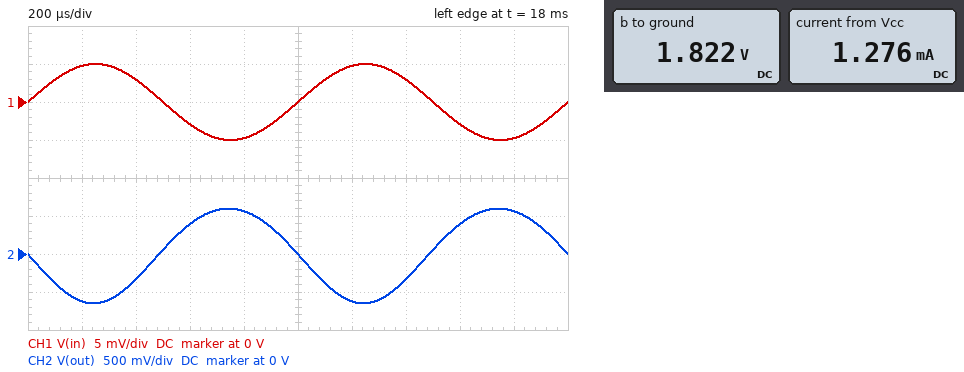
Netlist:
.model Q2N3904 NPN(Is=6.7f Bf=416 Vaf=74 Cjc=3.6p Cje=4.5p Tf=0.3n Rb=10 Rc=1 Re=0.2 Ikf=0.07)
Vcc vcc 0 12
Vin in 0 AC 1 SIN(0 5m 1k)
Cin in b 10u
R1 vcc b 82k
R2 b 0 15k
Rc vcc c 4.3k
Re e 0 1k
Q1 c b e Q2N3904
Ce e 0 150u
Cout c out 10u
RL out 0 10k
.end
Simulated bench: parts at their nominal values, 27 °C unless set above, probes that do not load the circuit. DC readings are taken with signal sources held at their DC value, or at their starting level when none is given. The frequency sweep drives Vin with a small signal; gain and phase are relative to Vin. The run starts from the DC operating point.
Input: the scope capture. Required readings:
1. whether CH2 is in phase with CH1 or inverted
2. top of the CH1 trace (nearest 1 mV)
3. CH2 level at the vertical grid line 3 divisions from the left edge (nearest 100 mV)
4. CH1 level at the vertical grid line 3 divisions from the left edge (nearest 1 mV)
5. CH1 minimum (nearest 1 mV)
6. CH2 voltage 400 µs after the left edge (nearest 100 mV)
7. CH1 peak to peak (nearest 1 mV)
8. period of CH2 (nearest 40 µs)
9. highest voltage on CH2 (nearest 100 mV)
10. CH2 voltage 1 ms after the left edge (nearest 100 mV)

inverted
5 mV
400 mV
-3 mV
-5 mV
-300 mV
10 mV
1.00 ms
600 mV
0 V
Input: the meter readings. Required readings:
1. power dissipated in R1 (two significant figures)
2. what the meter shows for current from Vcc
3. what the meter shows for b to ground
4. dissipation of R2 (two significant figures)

1.3 mW
1.276 mA
1.822 V
220 µW
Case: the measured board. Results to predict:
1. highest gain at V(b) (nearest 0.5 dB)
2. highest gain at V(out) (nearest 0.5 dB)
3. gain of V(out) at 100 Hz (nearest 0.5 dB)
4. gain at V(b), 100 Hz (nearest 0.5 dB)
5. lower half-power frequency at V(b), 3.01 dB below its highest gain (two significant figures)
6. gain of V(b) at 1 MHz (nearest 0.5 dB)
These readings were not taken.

0 dB
42.0 dB
41.0 dB
0 dB
1.3 Hz
0 dB
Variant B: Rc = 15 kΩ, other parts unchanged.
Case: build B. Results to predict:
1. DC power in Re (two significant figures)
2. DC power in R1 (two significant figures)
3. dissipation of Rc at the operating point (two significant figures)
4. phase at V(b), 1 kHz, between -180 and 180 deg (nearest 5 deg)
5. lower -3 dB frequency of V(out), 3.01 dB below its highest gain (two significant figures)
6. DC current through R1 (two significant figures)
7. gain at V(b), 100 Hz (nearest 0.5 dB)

600 µW
1.4 mW
8.3 mW
10 deg
220 Hz
130 µA
-7.5 dB
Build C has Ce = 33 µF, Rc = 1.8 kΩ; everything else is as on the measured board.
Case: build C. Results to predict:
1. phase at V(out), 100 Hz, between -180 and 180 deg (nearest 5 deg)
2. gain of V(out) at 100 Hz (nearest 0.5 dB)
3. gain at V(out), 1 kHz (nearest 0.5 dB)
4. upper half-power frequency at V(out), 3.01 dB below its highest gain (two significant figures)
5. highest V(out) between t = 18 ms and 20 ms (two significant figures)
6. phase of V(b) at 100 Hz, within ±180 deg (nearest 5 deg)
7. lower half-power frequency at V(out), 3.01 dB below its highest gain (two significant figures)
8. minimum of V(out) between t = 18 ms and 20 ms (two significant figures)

-115 deg
29.0 dB
36.0 dB
45 MHz
300 mV
0 deg
210 Hz
-330 mV
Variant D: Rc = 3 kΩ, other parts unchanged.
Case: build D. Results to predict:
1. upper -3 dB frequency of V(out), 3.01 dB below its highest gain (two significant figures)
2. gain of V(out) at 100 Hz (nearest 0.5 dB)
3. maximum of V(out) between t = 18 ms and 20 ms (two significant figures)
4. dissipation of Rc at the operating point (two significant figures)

29 MHz
39.0 dB
460 mV
4.0 mW
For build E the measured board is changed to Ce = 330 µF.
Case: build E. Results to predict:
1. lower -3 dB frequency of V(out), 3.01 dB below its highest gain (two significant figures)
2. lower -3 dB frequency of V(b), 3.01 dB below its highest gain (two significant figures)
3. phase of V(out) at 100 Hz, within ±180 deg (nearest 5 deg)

22 Hz
1.4 Hz
-165 deg
